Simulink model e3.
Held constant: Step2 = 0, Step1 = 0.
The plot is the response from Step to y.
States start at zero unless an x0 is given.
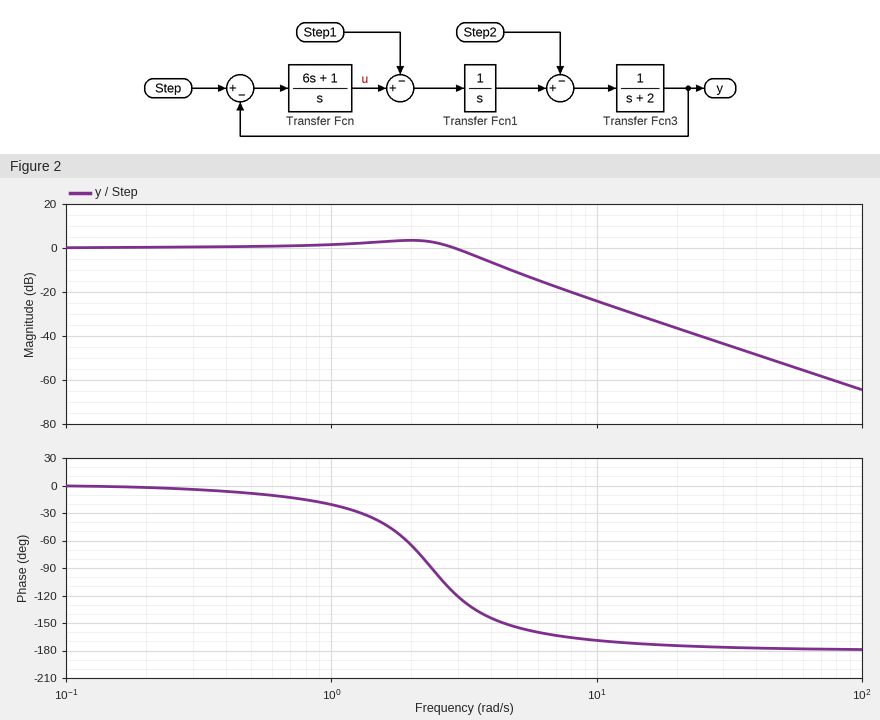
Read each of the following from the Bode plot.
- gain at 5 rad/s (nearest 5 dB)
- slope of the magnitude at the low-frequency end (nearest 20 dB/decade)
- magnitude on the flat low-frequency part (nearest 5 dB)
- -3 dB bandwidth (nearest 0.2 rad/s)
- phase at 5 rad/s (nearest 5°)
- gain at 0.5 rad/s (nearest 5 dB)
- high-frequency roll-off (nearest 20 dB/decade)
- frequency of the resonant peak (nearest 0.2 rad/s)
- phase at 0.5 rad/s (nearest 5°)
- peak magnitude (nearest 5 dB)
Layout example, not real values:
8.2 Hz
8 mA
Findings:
-10 dB
0 dB/decade
0 dB
3.4 rad/s
-155°
0 dB
-40 dB/decade
2.0 rad/s
-10°
5 dB
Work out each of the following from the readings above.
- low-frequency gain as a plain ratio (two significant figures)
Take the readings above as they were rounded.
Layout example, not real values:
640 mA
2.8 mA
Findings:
1.0
